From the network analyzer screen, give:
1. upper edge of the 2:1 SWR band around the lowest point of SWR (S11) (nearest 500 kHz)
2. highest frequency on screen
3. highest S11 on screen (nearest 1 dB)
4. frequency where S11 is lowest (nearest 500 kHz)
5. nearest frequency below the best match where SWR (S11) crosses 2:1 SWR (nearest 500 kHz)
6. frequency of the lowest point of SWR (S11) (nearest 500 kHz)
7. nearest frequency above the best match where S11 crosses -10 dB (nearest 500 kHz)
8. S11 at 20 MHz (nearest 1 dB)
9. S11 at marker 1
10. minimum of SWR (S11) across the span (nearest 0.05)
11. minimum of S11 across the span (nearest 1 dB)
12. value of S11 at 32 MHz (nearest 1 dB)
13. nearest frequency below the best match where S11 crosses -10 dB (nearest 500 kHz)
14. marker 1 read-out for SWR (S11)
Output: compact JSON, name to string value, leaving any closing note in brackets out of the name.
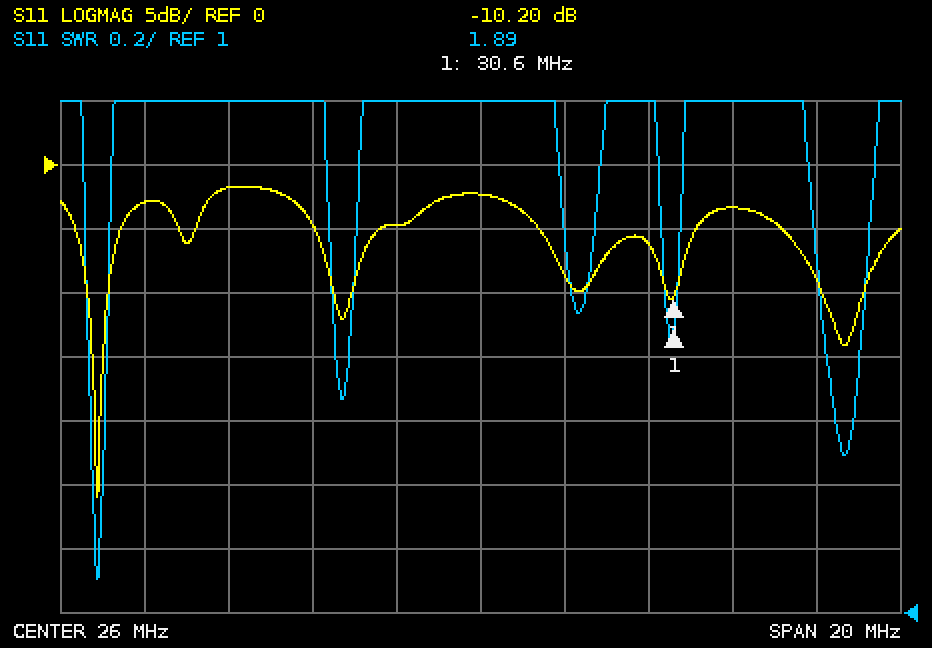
{"upper edge of the 2:1 SWR band around the lowest point of SWR (S11)": "17.0 MHz", "highest frequency on screen": "36 MHz", "highest S11 on screen": "-2 dB", "frequency where S11 is lowest": "17.0 MHz", "nearest frequency below the best match where SWR (S11) crosses 2:1 SWR": "16.5 MHz", "frequency of the lowest point of SWR (S11)": "17.0 MHz", "nearest frequency above the best match where S11 crosses -10 dB": "17.0 MHz", "S11 at 20 MHz": "-2 dB", "S11 at marker 1": "-10.20 dB", "minimum of SWR (S11) across the span": "1.10", "minimum of S11 across the span": "-26 dB", "value of S11 at 32 MHz": "-3 dB", "nearest frequency below the best match where S11 crosses -10 dB": "16.5 MHz", "marker 1 read-out for SWR": "1.89"}
